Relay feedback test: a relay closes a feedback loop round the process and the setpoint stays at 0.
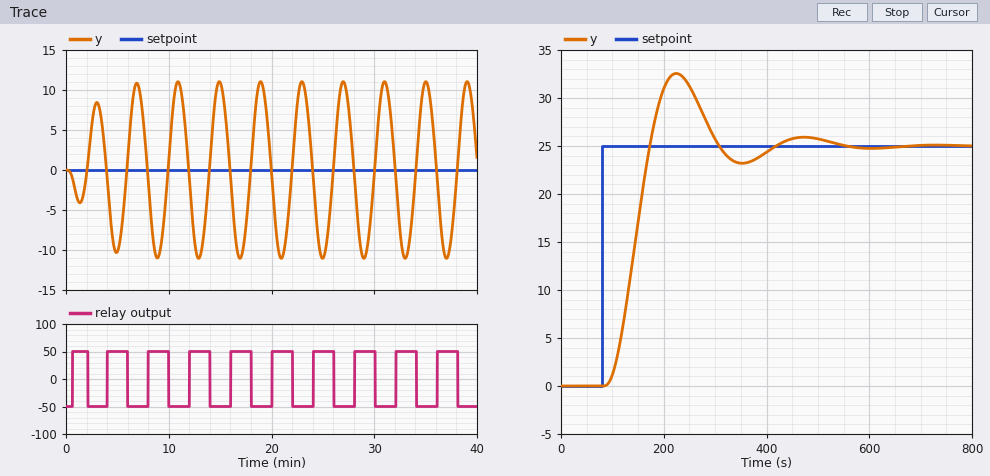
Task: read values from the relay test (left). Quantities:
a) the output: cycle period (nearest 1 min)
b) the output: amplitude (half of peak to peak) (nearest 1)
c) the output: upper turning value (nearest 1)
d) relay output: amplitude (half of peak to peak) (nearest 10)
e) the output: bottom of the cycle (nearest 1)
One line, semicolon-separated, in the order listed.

4 min; 11; 11; 50; -11
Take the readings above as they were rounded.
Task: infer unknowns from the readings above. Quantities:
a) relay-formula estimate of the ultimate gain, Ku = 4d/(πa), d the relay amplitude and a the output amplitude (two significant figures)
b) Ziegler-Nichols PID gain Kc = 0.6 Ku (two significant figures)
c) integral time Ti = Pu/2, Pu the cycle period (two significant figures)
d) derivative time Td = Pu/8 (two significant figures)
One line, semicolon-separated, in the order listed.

5.8; 3.5; 2.0 min; 0.50 min
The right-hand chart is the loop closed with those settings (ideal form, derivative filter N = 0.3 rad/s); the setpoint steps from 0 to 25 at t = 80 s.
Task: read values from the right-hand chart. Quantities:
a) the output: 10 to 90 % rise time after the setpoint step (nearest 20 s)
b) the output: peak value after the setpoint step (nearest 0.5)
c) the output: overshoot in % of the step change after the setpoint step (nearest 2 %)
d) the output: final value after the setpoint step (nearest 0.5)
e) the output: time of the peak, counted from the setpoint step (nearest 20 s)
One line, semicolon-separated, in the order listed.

60 s; 32.5; 30 %; 25.0; 140 s
